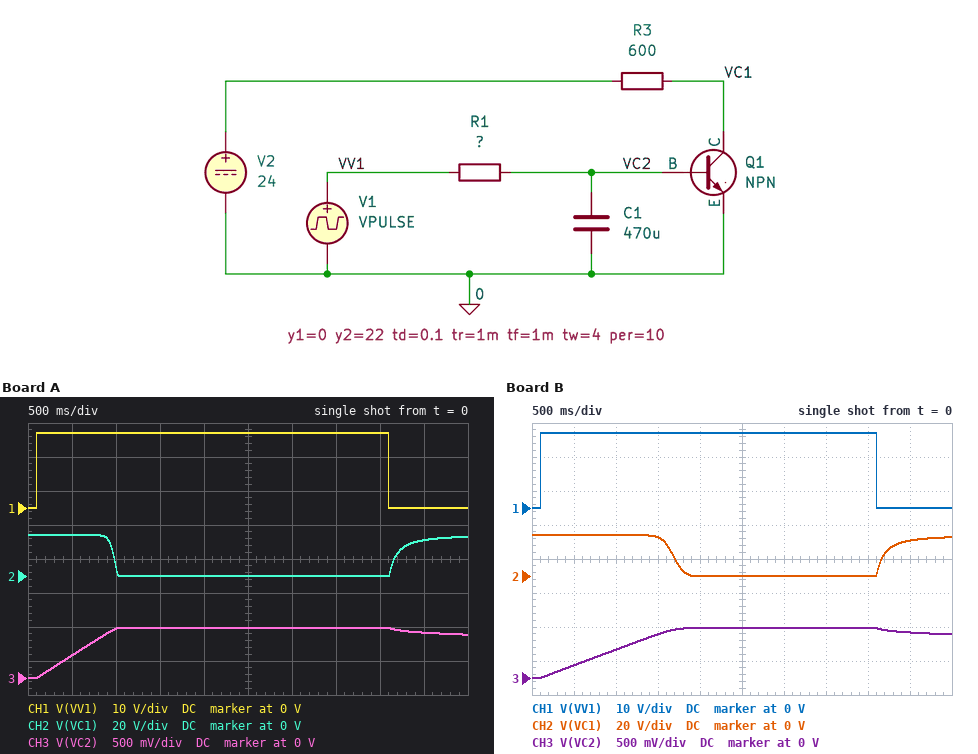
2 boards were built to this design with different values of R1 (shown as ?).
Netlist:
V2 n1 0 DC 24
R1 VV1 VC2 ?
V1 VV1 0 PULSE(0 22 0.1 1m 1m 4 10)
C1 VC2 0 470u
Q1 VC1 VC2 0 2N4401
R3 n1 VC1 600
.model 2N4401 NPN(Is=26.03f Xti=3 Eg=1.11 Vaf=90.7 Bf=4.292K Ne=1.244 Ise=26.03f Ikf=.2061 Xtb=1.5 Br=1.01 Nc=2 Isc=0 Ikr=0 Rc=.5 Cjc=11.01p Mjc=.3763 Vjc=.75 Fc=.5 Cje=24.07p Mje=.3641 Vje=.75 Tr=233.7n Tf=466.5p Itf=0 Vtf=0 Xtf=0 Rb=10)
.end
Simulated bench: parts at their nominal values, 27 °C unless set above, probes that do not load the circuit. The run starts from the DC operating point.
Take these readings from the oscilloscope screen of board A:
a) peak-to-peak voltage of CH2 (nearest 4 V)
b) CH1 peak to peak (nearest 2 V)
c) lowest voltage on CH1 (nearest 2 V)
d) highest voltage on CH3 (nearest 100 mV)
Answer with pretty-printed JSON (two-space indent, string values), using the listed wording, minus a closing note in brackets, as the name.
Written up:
{
  "peak-to-peak voltage of CH2": "24 V",
  "CH1 peak to peak": "22 V",
  "lowest voltage on CH1": "0 V",
  "highest voltage on CH3": "700 mV"
}
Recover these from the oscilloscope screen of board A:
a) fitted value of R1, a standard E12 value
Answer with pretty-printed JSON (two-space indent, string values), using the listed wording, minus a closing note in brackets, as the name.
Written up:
{
  "fitted value of R1, a standard E12 value": "56 kΩ"
}
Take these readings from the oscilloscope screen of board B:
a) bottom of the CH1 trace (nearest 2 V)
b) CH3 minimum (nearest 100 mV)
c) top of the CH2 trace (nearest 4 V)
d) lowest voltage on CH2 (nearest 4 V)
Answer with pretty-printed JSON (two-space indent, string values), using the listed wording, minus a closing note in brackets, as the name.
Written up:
{
  "bottom of the CH1 trace": "0 V",
  "CH3 minimum": "0 V",
  "top of the CH2 trace": "24 V",
  "lowest voltage on CH2": "0 V"
}
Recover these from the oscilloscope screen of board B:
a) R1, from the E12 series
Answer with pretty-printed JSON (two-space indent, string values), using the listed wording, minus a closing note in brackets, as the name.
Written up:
{
  "R1, from the E12 series": "100 kΩ"
}
